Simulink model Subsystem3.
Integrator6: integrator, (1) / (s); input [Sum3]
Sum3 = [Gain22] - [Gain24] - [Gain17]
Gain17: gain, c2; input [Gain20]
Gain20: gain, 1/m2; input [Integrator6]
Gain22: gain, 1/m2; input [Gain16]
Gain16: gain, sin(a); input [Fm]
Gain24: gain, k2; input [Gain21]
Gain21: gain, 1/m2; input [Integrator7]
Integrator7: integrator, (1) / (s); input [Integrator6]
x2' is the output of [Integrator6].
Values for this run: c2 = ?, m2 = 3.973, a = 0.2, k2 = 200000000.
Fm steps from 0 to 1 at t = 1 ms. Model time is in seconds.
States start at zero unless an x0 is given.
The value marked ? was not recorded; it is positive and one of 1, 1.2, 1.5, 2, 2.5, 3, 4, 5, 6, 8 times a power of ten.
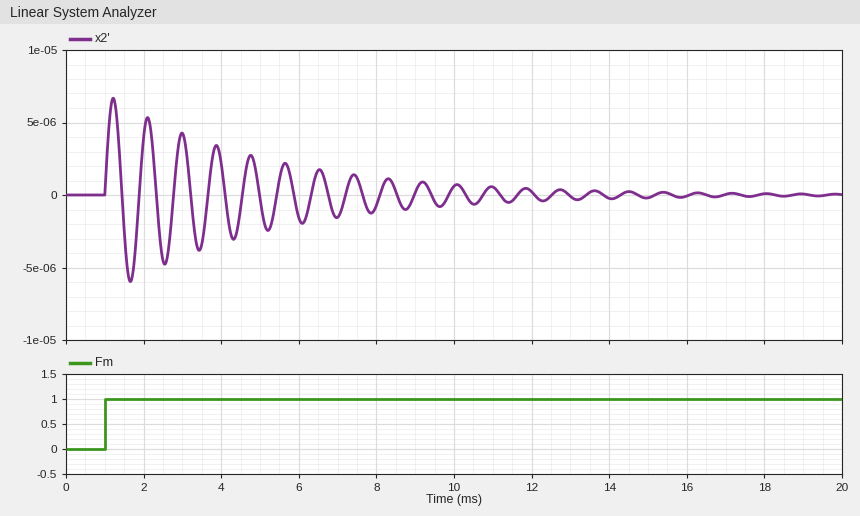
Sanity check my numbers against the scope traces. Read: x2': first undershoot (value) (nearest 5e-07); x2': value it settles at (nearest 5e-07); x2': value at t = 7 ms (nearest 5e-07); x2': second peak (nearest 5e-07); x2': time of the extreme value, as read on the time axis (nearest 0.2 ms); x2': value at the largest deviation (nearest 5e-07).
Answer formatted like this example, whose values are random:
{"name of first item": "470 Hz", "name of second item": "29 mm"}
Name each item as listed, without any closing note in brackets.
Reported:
{"x2': first undershoot (value)": "-0.0000060", "x2': value it settles at": "0.0000000", "x2': value at t = 7 ms": "-0.0000015", "x2': second peak": "0.0000055", "x2': time of the extreme value, as read on the time axis": "1.2 ms", "x2': value at the largest deviation": "0.0000065"}
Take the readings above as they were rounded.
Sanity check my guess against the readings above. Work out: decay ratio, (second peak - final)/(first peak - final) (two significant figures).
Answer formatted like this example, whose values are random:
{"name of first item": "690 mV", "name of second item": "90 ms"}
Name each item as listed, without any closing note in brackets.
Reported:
{"decay ratio, (second peak - final)/(first peak - final)": "0.85"}
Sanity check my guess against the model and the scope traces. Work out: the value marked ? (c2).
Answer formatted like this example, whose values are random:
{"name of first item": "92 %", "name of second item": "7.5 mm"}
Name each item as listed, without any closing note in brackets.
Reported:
{"the value marked ?": "2000"}
